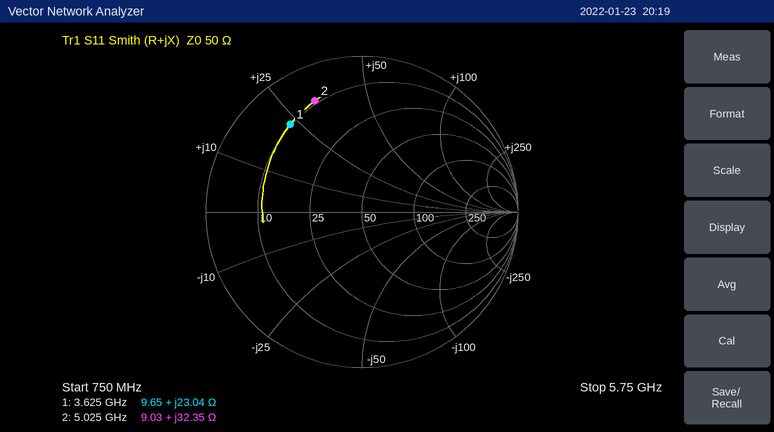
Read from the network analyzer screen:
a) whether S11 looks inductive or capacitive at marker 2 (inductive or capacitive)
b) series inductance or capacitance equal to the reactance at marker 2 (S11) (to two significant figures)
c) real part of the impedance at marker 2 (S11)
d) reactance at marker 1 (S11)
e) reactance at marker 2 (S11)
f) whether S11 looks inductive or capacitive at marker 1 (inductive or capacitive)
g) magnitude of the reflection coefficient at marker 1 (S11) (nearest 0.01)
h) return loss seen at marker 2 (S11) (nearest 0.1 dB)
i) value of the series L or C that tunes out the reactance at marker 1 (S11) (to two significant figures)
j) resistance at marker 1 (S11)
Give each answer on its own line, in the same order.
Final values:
inductive
1.0 nH
9.03 Ω
+23.04 Ω
+32.35 Ω
inductive
0.73
2.2 dB
1.9 pF
9.65 Ω
